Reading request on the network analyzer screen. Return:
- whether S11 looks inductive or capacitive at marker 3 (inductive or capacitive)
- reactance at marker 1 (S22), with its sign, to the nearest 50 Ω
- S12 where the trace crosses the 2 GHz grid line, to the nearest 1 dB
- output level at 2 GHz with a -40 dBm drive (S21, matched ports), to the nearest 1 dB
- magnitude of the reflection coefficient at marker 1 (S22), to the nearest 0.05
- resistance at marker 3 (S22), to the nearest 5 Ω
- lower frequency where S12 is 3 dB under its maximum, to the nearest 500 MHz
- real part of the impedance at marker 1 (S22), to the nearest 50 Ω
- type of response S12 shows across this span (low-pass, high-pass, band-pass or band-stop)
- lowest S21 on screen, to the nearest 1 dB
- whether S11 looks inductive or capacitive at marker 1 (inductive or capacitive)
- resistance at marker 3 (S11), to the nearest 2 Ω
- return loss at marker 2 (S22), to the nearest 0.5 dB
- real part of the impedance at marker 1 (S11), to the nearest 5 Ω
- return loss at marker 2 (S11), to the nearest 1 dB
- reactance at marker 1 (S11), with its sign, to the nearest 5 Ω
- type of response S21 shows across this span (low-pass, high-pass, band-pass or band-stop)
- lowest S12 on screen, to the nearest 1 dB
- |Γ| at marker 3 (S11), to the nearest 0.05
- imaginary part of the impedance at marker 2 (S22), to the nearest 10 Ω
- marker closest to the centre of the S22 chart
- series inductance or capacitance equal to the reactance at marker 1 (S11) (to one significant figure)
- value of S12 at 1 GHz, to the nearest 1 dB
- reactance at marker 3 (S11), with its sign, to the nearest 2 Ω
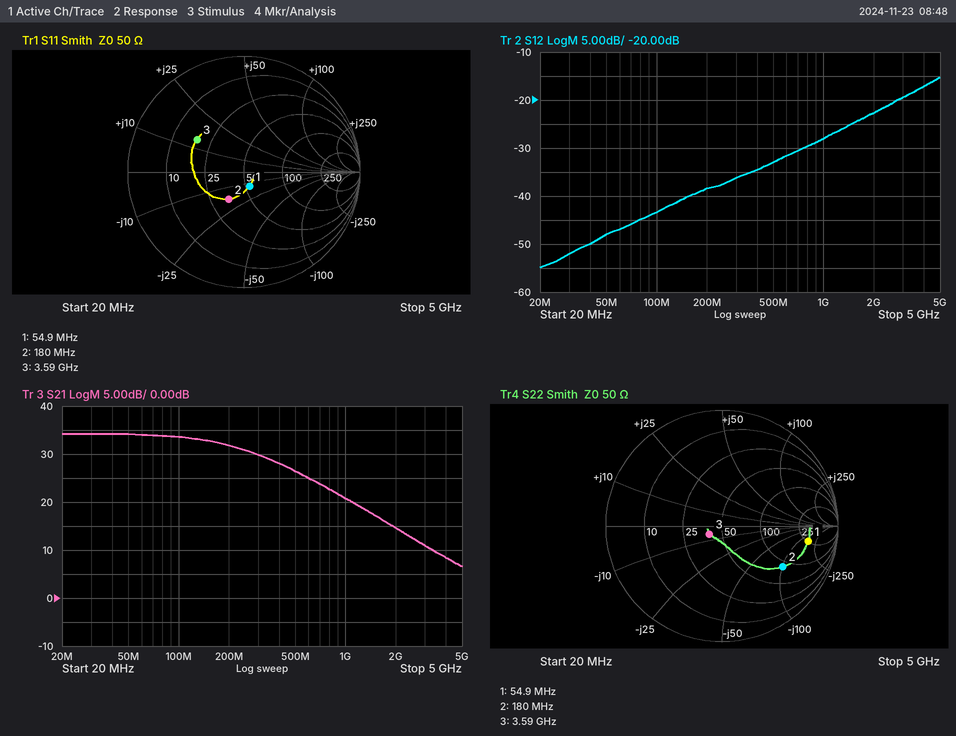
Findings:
inductive
-150 Ω
-23 dB
-25 dBm
0.75
40 Ω
3.5 GHz
250 Ω
high-pass
7 dB
capacitive
18 Ω
4.0 dB
55 Ω
11 dB
-15 Ω
low-pass
-55 dB
0.50
-100 Ω
marker 3
200 pF
-28 dB
+14 Ω
